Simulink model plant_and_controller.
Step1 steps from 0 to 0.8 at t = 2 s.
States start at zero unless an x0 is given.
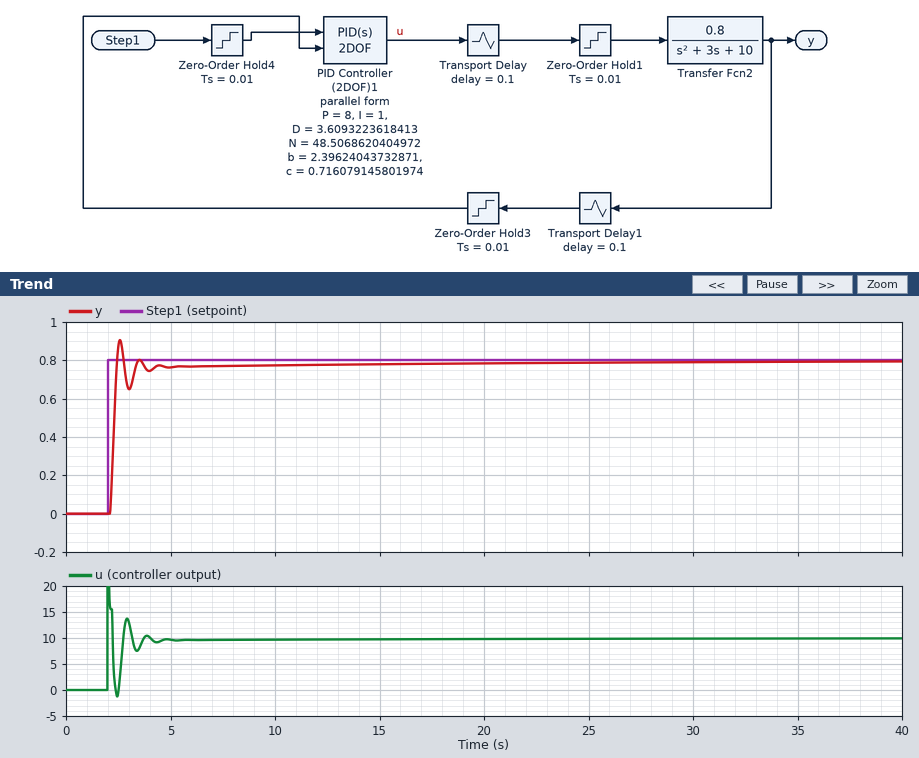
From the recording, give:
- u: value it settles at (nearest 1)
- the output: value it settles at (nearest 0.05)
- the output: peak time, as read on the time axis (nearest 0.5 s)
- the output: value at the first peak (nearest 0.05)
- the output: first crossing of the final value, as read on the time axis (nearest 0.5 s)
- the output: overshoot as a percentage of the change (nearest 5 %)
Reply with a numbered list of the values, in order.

1. 10
2. 0.80
3. 2.5 s
4. 0.90
5. 2.5 s
6. 15 %
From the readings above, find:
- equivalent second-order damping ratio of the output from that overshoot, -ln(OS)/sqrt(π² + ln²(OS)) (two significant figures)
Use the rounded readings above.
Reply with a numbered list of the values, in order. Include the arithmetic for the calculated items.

1. ln(0.15) = -1.897; 1.897 / sqrt(9.870 + 3.599) = 0.52
